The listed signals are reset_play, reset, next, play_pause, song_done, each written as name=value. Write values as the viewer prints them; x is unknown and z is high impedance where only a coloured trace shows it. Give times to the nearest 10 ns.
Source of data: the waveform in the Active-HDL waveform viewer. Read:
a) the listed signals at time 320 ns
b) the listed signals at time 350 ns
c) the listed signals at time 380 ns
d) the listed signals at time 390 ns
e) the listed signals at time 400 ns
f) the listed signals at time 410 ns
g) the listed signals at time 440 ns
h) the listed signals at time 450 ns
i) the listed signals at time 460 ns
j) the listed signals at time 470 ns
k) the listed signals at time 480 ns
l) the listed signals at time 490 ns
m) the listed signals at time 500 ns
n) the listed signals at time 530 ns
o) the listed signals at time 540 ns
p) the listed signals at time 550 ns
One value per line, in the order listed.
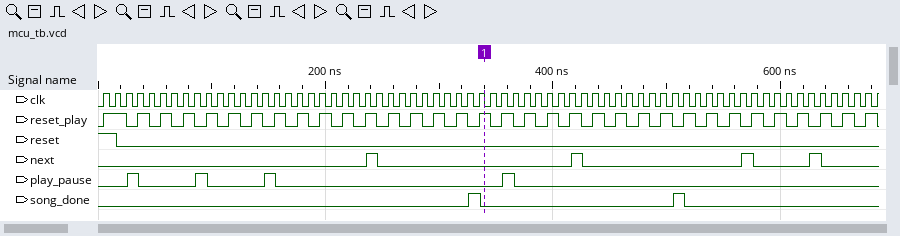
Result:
reset_play=1, reset=0, next=0, play_pause=0, song_done=0
reset_play=0, reset=0, next=0, play_pause=0, song_done=0
reset_play=1, reset=0, next=0, play_pause=0, song_done=0
reset_play=0, reset=0, next=0, play_pause=0, song_done=0
reset_play=1, reset=0, next=0, play_pause=0, song_done=0
reset_play=0, reset=0, next=0, play_pause=0, song_done=0
reset_play=1, reset=0, next=0, play_pause=0, song_done=0
reset_play=0, reset=0, next=0, play_pause=0, song_done=0
reset_play=1, reset=0, next=0, play_pause=0, song_done=0
reset_play=0, reset=0, next=0, play_pause=0, song_done=0
reset_play=1, reset=0, next=0, play_pause=0, song_done=0
reset_play=0, reset=0, next=0, play_pause=0, song_done=0
reset_play=1, reset=0, next=0, play_pause=0, song_done=0
reset_play=0, reset=0, next=0, play_pause=0, song_done=0
reset_play=1, reset=0, next=0, play_pause=0, song_done=0
reset_play=0, reset=0, next=0, play_pause=0, song_done=0
